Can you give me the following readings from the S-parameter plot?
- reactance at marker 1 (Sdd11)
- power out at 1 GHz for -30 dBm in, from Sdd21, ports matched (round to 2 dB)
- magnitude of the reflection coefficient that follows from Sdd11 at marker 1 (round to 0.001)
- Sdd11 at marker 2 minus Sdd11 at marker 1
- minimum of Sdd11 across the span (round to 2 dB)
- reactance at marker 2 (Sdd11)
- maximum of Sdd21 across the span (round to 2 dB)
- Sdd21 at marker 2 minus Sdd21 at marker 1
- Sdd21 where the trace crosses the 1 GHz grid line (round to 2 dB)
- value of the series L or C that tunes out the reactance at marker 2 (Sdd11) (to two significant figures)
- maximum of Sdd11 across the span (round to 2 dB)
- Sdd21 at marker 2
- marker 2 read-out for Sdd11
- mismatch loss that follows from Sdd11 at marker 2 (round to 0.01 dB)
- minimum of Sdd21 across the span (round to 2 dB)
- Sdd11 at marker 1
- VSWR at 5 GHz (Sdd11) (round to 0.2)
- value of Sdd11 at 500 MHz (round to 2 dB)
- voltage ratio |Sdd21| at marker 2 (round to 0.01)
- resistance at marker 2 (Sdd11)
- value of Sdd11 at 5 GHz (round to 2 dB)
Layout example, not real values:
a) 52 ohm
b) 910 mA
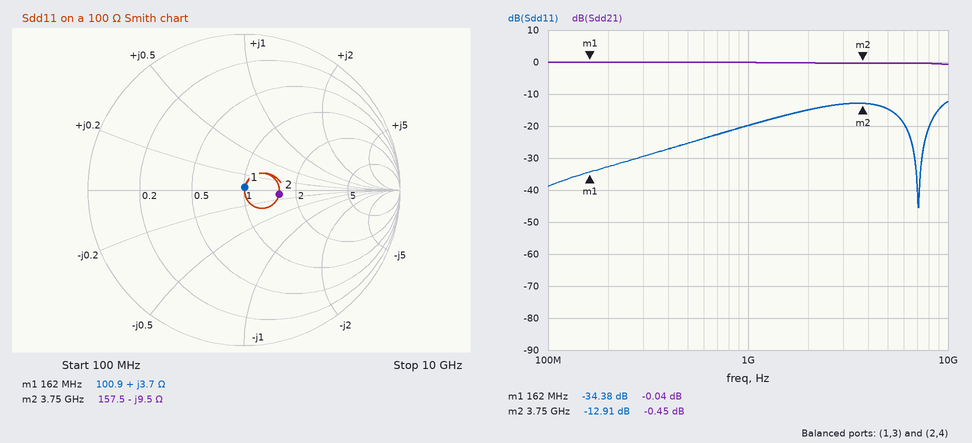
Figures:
a) +3.7 Ω
b) -30 dBm
c) 0.019
d) 21.47 dB
e) -46 dB
f) -9.5 Ω
g) 0 dB
h) -0.41 dB
i) 0 dB
j) 400 pH
k) -12 dB
l) -0.45 dB
m) -12.91 dB
n) 0.23 dB
o) 0 dB
p) -34.38 dB
q) 1.4
r) -26 dB
s) 0.95
t) 157.5 Ω
u) -14 dB
